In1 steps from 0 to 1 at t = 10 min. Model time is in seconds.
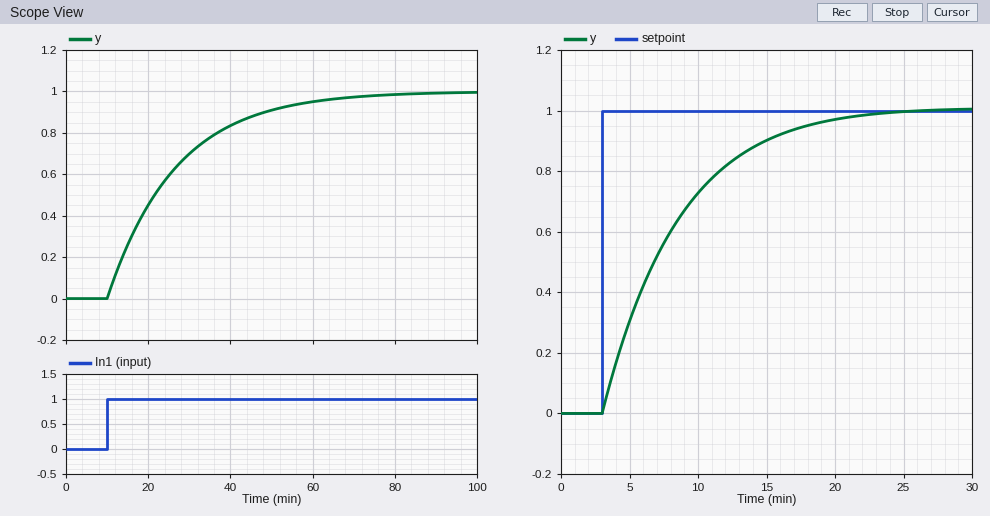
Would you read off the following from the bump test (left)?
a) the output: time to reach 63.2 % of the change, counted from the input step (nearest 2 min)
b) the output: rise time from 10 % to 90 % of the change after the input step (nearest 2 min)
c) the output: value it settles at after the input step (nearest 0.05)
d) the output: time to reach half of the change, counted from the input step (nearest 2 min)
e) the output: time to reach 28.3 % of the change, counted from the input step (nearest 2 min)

16 min
36 min
1.00
12 min
6 min
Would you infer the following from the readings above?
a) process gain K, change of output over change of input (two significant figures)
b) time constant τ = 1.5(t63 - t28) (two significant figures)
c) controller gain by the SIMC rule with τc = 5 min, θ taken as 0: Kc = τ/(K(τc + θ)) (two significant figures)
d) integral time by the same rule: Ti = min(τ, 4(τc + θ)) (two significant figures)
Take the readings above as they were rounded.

1.0
15 min
3.0
15 min
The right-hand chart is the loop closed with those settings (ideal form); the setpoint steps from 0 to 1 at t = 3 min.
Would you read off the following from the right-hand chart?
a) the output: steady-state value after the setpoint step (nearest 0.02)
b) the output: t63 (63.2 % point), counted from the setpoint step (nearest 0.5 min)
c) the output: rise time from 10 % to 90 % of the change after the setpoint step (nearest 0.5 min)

1.00
5.5 min
11.5 min
